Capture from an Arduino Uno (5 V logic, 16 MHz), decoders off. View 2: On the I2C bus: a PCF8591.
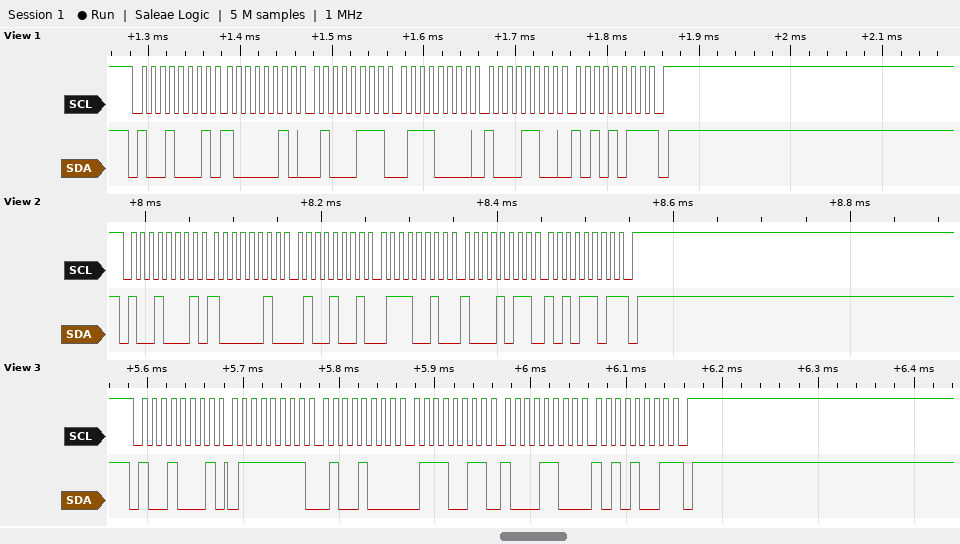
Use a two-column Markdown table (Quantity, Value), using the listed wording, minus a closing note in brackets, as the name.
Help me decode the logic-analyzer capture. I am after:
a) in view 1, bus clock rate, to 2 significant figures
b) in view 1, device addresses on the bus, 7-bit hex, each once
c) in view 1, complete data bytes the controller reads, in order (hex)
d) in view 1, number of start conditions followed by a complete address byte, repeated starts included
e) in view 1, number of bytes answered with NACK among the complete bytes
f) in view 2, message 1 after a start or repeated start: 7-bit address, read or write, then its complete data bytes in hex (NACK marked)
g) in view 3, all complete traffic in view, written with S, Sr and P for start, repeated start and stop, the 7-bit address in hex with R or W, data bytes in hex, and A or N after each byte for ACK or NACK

| Quantity | Value |
|---|---|
| in view 1, bus clock rate, to 2 significant figures | 100 kHz |
| in view 1, device addresses on the bus, 7-bit hex, each once | 0x48 |
| in view 1, complete data bytes the controller reads, in order | 82 47 70 8C AB |
| in view 1, number of start conditions followed by a complete address byte, repeated starts included | 1 |
| in view 1, number of bytes answered with NACK among the complete bytes | 1 |
| in view 2, message 1 after a start or repeated start: 7-bit address, read or write, then its complete data bytes in hex | 0x48 read: 82 49 72 8B AD NACK |
| in view 3, all complete traffic in view, written with S, Sr and P for start, repeated start and stop, the 7-bit address in hex with R or W, data bytes in hex, and A or N after each byte for ACK or NACK | S 48R A 7F A 48 A 73 A 8C A A9 N P |
